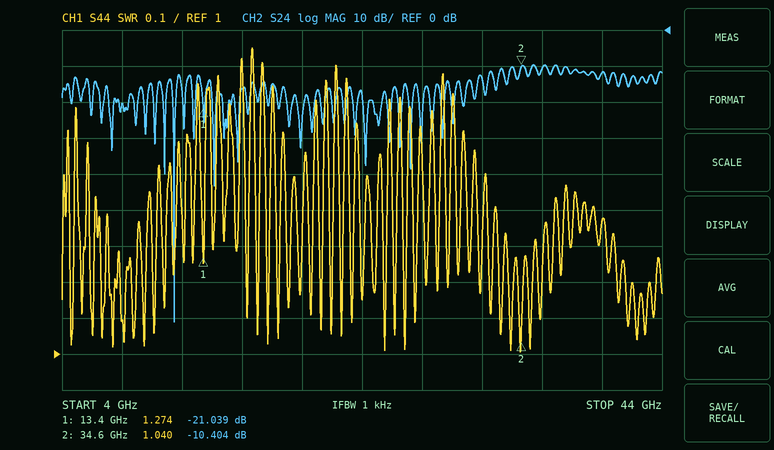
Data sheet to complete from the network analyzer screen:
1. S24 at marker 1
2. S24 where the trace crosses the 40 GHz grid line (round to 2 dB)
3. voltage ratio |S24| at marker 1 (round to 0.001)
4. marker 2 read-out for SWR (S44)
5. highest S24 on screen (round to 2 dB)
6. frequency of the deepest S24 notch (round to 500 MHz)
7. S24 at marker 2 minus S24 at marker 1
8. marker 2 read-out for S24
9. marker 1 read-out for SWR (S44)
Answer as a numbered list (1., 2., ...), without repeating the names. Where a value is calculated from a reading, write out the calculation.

1. -21.039 dB
2. -12 dB
3. 10^(-21.039/20) ≈ 0.089
4. 1.040
5. -10 dB
6. 11.5 GHz
7. -10.404 − (-21.039) = 10.635 dB
8. -10.404 dB
9. 1.274
